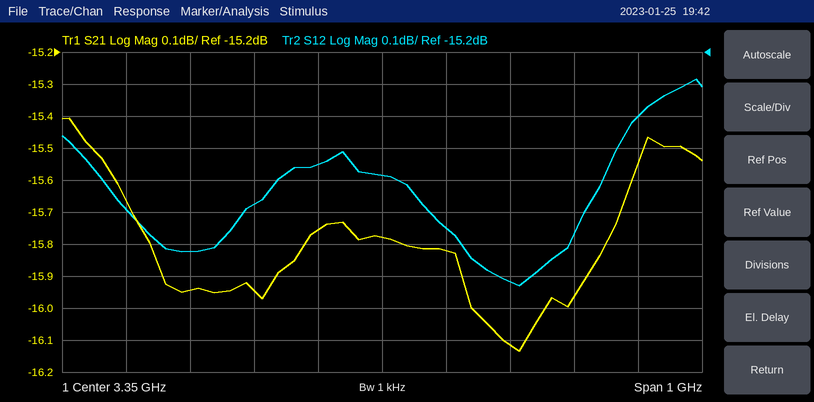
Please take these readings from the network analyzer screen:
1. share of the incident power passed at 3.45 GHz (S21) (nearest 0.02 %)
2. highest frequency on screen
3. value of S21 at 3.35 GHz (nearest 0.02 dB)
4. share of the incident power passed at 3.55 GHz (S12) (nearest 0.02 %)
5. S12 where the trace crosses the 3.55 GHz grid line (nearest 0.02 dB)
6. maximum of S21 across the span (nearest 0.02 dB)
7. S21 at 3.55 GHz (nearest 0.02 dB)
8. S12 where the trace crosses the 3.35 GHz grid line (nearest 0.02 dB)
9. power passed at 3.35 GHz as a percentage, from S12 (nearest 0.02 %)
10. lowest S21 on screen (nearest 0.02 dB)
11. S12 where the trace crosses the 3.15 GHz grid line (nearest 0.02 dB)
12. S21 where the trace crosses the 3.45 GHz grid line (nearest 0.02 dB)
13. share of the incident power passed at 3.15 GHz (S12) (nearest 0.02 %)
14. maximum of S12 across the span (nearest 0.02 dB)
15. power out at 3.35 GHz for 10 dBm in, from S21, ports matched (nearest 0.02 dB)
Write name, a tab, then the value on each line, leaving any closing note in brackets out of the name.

share of the incident power passed at 3.45 GHz (S21)	2.62 %
highest frequency on screen	3.85 GHz
value of S21 at 3.35 GHz	-15.78 dB
share of the incident power passed at 3.55 GHz (S12)	2.56 %
S12 where the trace crosses the 3.55 GHz grid line	-15.92 dB
maximum of S21 across the span	-15.40 dB
S21 at 3.55 GHz	-16.12 dB
S12 where the trace crosses the 3.35 GHz grid line	-15.58 dB
power passed at 3.35 GHz as a percentage, from S12	2.76 %
lowest S21 on screen	-16.14 dB
S12 where the trace crosses the 3.15 GHz grid line	-15.68 dB
S21 where the trace crosses the 3.45 GHz grid line	-15.82 dB
share of the incident power passed at 3.15 GHz (S12)	2.70 %
maximum of S12 across the span	-15.28 dB
power out at 3.35 GHz for 10 dBm in, from S21, ports matched	-5.78 dBm
